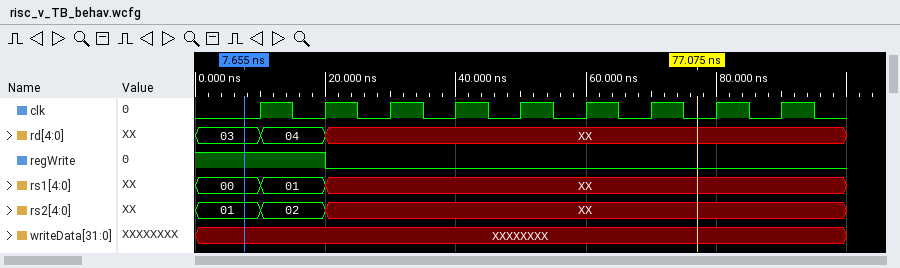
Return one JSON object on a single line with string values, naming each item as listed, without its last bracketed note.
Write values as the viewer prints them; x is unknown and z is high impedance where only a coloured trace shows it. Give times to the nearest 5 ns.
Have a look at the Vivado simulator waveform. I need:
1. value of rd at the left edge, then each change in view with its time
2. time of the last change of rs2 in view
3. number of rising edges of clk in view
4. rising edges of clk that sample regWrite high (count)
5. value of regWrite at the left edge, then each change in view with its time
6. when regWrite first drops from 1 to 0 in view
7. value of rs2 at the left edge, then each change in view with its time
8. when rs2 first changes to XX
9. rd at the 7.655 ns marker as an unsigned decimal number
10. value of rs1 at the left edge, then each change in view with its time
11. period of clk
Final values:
{"value of rd at the left edge, then each change in view with its time": "03, 04 at 10 ns, XX at 20 ns", "time of the last change of rs2 in view": "20 ns", "number of rising edges of clk in view": "9", "rising edges of clk that sample regWrite high": "2", "value of regWrite at the left edge, then each change in view with its time": "1, 0 at 20 ns", "when regWrite first drops from 1 to 0 in view": "20 ns", "value of rs2 at the left edge, then each change in view with its time": "01, 02 at 10 ns, XX at 20 ns", "when rs2 first changes to XX": "20 ns", "rd at the 7.655 ns marker as an unsigned decimal number": "3", "value of rs1 at the left edge, then each change in view with its time": "00, 01 at 10 ns, XX at 20 ns", "period of clk": "10 ns"}
